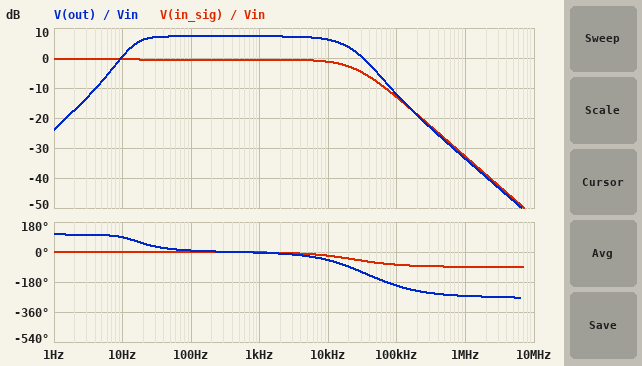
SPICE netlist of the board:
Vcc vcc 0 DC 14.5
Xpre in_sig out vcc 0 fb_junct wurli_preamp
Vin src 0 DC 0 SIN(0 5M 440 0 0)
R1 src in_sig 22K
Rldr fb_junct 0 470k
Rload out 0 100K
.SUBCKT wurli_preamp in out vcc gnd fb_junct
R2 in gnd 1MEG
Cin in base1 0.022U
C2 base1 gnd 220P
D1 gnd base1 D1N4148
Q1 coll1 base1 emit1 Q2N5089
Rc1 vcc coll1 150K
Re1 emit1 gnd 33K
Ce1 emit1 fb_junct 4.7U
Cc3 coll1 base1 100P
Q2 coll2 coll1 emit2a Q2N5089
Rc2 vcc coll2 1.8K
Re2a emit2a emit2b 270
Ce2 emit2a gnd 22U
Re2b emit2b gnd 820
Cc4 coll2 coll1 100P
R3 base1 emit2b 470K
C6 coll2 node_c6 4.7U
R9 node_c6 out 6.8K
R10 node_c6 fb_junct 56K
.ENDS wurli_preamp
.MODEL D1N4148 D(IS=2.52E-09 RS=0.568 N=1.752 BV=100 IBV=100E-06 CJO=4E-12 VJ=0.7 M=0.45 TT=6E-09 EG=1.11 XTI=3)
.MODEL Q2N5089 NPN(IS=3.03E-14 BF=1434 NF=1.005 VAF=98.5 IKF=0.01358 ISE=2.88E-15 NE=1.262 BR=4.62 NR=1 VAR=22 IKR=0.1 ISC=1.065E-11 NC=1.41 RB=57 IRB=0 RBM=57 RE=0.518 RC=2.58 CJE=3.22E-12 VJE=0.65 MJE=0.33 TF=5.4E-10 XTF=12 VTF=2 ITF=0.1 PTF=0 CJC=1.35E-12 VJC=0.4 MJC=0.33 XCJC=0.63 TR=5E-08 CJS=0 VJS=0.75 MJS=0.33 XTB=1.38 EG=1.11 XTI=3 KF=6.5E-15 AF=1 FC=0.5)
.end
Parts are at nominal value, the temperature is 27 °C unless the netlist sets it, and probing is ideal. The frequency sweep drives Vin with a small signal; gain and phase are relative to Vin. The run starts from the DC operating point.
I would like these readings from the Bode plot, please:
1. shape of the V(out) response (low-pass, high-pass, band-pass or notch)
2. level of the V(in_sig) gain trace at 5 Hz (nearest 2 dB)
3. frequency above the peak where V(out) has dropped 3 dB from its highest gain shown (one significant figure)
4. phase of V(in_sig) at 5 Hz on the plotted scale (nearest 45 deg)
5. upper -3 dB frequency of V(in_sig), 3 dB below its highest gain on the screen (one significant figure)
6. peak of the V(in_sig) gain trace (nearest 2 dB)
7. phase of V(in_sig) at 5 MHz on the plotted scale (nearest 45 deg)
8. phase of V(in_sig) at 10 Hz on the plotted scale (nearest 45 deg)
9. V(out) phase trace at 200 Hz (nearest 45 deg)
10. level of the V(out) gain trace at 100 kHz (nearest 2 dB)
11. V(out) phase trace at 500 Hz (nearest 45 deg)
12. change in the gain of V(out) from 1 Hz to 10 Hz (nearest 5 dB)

band-pass
0 dB
20 kHz
0 deg
20 kHz
0 dB
-90 deg
0 deg
0 deg
-12 dB
0 deg
25 dB
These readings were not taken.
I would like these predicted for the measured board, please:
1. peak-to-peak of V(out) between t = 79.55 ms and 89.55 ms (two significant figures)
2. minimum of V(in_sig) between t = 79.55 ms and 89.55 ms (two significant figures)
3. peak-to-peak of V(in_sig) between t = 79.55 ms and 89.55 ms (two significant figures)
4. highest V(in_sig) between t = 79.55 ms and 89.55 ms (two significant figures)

23 mV
-4.7 mV
9.4 mV
4.7 mV
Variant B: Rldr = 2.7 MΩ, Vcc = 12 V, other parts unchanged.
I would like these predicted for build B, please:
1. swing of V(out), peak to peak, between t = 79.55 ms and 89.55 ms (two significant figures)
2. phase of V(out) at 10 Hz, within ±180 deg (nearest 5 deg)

22 mV
85 deg
